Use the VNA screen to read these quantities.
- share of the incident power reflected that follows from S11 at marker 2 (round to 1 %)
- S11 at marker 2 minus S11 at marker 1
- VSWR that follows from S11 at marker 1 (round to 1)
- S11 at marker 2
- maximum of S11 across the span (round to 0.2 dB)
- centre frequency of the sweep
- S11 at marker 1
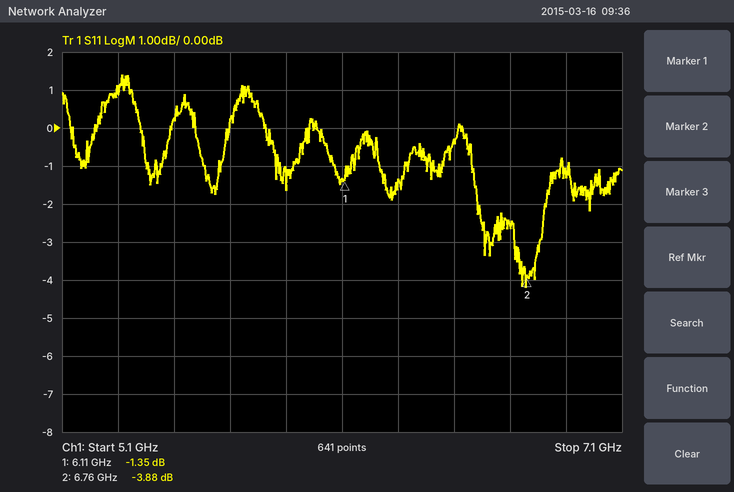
41 %
-2.53 dB
13
-3.88 dB
1.4 dB
6.1 GHz
-1.35 dB
